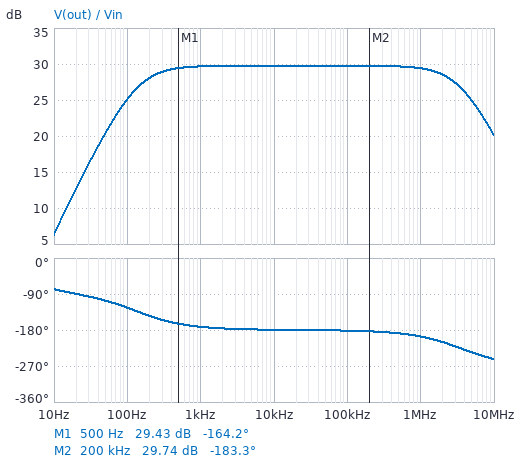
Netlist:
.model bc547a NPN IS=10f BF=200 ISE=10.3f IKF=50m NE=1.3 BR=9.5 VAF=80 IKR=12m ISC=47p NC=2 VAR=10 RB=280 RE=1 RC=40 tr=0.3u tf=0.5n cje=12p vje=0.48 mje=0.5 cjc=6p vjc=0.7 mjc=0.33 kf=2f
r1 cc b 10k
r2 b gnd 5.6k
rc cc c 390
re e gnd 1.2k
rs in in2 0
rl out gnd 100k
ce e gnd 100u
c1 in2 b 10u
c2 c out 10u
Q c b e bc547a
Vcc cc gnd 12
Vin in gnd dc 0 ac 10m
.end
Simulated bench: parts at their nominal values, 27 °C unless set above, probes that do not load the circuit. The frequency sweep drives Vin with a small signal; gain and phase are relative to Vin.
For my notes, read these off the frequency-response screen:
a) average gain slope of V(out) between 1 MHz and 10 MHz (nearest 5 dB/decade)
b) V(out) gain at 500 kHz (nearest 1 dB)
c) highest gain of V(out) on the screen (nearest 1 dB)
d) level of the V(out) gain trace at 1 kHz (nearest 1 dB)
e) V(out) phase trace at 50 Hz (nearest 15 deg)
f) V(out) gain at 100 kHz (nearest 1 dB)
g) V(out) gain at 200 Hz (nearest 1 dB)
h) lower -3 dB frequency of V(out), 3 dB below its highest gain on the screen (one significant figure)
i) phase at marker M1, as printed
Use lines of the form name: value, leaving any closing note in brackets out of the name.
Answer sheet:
average gain slope of V(out) between 1 MHz and 10 MHz: -10 dB/decade
V(out) gain at 500 kHz: 30 dB
highest gain of V(out) on the screen: 30 dB
level of the V(out) gain trace at 1 kHz: 30 dB
V(out) phase trace at 50 Hz: -105 deg
V(out) gain at 100 kHz: 30 dB
V(out) gain at 200 Hz: 28 dB
lower -3 dB frequency of V(out), 3 dB below its highest gain on the screen: 100 Hz
phase at marker M1, as printed: -164.2 deg
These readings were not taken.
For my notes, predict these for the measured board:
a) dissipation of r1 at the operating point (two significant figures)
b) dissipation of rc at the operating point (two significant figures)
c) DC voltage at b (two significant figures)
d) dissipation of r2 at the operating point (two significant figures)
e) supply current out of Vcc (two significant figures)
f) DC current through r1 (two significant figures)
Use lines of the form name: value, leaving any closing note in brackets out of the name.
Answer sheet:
dissipation of r1 at the operating point: 6.0 mW
dissipation of rc at the operating point: 3.3 mW
DC voltage at b: 4.2 V
dissipation of r2 at the operating point: 3.2 mW
supply current out of Vcc: 3.7 mA
DC current through r1: 780 µA
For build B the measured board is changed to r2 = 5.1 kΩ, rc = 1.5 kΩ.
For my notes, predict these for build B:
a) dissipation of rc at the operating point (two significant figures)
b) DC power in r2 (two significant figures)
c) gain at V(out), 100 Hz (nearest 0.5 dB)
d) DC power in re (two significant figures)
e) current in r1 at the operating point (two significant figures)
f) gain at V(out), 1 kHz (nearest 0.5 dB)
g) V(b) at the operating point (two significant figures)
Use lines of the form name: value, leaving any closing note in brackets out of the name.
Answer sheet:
dissipation of rc at the operating point: 11 mW
DC power in r2: 3.1 mW
gain at V(out), 100 Hz: 36.5 dB
DC power in re: 9.0 mW
current in r1 at the operating point: 800 µA
gain at V(out), 1 kHz: 40.5 dB
V(b) at the operating point: 4.0 V
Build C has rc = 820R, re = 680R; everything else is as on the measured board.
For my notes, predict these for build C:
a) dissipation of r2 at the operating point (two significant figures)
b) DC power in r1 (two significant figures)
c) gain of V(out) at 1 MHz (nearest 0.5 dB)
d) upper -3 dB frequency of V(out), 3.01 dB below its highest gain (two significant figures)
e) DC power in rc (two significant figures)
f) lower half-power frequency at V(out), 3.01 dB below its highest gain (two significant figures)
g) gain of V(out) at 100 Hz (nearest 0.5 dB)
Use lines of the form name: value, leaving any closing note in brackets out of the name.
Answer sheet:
dissipation of r2 at the operating point: 3.1 mW
DC power in r1: 6.1 mW
gain of V(out) at 1 MHz: 37.0 dB
upper -3 dB frequency of V(out), 3.01 dB below its highest gain: 1.5 MHz
DC power in rc: 21 mW
lower half-power frequency at V(out), 3.01 dB below its highest gain: 190 Hz
gain of V(out) at 100 Hz: 32.0 dB
